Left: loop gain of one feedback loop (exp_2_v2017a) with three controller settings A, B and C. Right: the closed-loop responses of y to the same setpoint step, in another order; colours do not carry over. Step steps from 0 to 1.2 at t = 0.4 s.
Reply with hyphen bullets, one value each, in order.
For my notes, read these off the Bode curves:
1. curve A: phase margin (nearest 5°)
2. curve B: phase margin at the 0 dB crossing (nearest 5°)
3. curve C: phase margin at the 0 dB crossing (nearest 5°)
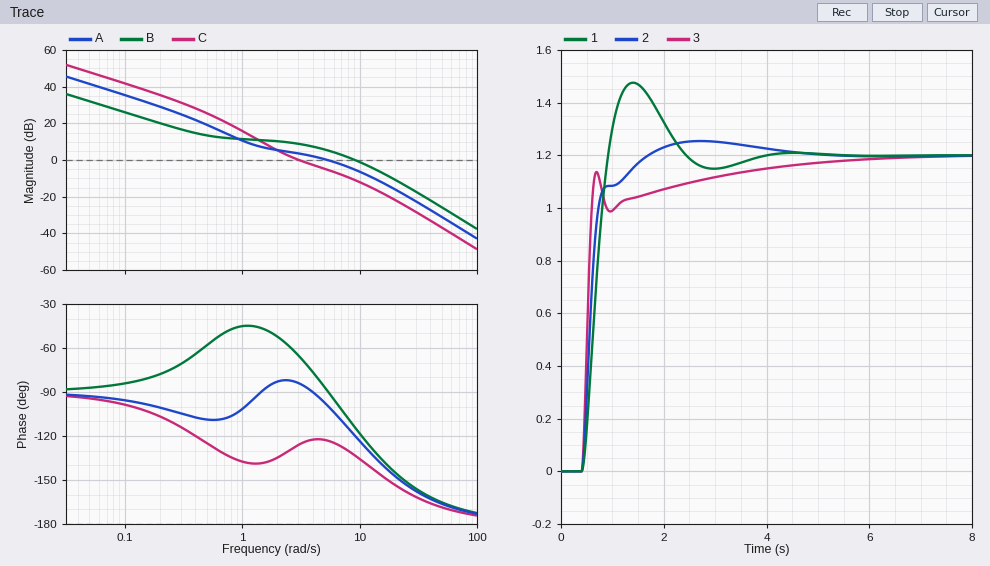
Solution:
- 80°
- 65°
- 55°
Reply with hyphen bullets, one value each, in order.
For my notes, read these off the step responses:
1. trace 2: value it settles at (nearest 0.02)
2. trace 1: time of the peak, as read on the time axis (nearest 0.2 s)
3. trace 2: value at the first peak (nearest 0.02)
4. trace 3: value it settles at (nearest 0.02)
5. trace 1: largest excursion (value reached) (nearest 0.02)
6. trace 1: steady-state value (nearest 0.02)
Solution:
- 1.20
- 1.4 s
- 1.26
- 1.20
- 1.48
- 1.20
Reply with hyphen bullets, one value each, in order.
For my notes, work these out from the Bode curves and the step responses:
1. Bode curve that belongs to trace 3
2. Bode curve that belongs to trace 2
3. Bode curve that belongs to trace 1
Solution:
- B
- A
- C
